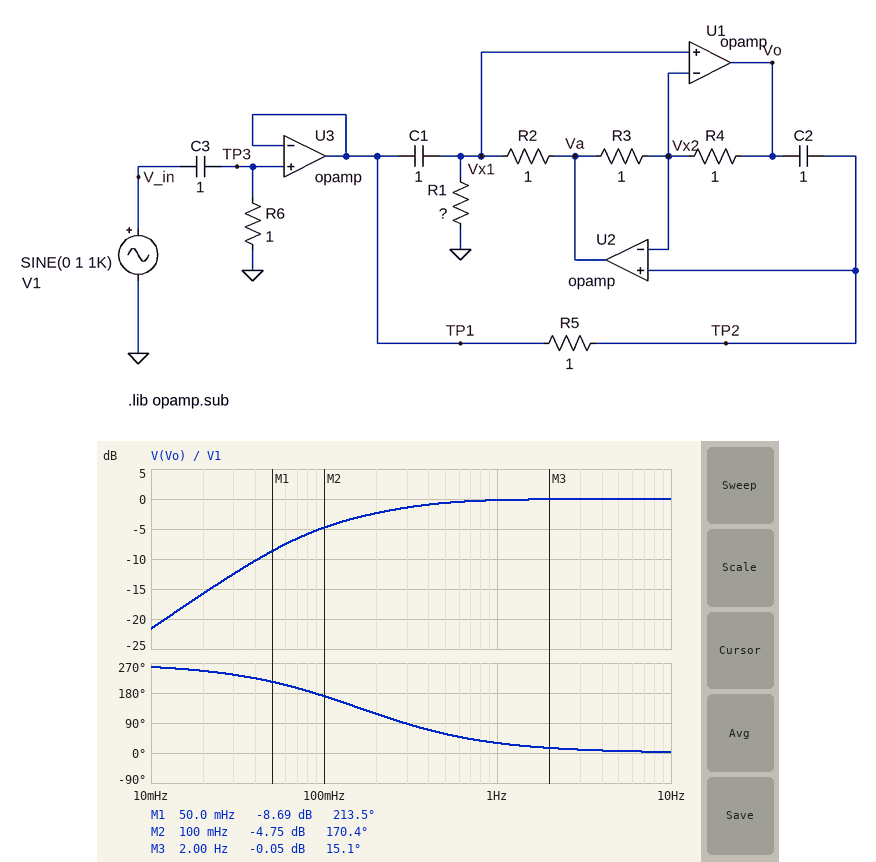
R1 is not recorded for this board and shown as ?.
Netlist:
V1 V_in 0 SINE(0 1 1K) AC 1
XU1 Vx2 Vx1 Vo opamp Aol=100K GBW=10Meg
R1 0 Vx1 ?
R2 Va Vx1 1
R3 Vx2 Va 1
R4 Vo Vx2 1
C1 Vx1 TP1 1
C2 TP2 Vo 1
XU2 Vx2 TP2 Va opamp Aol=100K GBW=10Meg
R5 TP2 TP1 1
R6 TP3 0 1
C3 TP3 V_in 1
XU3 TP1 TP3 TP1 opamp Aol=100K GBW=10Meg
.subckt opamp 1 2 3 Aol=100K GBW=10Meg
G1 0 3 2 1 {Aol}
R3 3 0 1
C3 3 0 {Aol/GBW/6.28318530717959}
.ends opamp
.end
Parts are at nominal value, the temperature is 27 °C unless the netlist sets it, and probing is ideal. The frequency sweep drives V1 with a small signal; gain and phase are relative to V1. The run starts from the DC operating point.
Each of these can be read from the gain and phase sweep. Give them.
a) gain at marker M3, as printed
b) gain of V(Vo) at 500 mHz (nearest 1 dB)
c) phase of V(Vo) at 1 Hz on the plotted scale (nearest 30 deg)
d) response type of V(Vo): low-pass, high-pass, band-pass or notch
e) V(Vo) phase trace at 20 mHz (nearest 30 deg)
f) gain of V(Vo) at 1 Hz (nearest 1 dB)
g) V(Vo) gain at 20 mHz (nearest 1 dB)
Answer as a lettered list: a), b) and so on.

a) -0.05 dB
b) -1 dB
c) 30 deg
d) high-pass
e) 240 deg
f) 0 dB
g) -16 dB
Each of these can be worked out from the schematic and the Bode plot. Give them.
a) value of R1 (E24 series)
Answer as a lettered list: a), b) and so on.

a) 0.43 Ω
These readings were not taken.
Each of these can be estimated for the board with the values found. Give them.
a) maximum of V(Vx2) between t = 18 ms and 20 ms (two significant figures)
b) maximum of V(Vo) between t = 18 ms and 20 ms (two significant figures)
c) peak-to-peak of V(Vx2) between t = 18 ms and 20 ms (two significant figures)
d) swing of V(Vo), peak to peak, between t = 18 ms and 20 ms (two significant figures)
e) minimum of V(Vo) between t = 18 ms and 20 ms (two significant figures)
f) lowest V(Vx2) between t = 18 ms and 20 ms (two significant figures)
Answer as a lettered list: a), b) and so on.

a) 1.0 V
b) 1.0 V
c) 2.0 V
d) 2.0 V
e) -1.0 V
f) -1.0 V
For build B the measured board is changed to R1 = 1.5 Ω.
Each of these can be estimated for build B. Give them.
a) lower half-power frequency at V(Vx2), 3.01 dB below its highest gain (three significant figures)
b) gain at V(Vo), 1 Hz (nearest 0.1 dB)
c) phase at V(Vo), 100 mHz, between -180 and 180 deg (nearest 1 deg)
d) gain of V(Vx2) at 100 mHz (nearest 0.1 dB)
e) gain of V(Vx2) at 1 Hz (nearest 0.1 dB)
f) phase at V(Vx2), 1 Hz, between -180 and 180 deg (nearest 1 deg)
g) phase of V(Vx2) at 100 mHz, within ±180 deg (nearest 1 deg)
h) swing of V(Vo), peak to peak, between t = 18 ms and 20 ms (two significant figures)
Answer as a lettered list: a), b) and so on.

a) 257 mHz
b) 0 dB
c) -157 deg
d) -7.2 dB
e) -0.2 dB
f) 15 deg
g) 23 deg
h) 2.0 V
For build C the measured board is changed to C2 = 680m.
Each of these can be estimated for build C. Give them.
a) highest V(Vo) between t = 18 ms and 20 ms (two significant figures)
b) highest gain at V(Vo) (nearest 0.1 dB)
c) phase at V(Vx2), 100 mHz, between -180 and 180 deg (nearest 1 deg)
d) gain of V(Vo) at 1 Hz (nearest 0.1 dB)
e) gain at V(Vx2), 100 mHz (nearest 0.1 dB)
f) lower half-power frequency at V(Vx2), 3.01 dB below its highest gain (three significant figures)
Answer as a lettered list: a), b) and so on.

a) 1.0 V
b) 0.1 dB
c) 4 deg
d) 0 dB
e) -10.0 dB
f) 488 mHz
